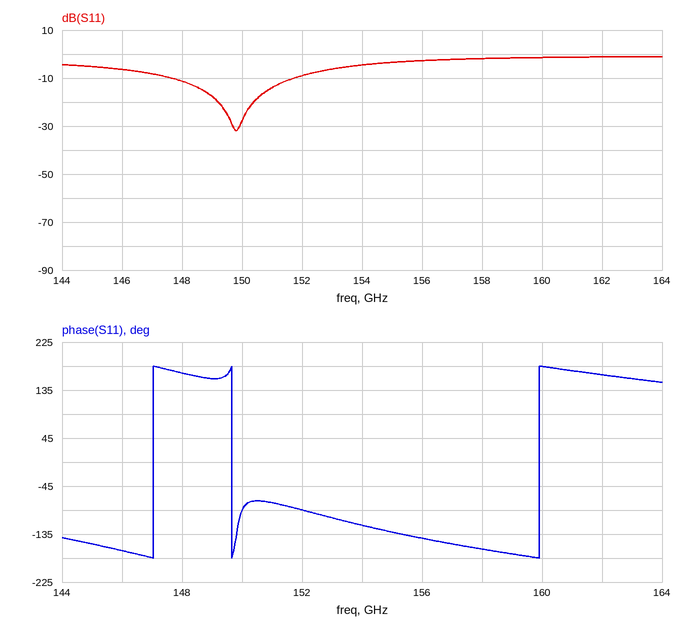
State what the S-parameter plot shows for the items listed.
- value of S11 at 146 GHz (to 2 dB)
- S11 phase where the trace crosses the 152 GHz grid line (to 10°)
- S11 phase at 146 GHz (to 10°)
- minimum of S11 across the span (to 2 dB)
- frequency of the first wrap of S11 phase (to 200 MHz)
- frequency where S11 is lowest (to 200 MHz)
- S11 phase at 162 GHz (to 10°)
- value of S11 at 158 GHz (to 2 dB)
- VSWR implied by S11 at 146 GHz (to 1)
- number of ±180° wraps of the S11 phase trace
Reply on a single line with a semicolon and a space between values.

-6 dB; -90°; -170°; -32 dB; 147.0 GHz; 149.8 GHz; 160°; -2 dB; 3; 3
